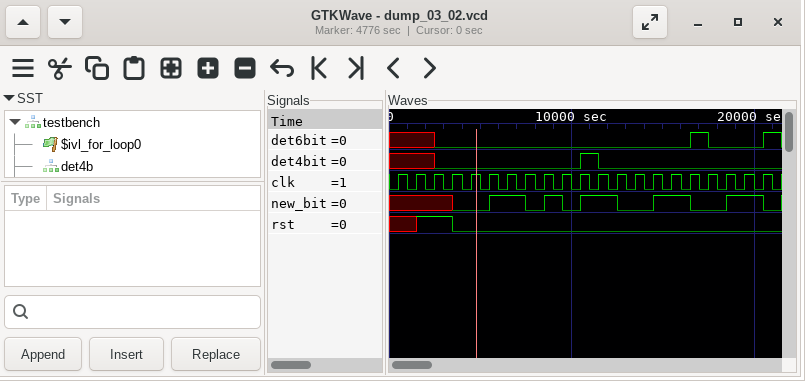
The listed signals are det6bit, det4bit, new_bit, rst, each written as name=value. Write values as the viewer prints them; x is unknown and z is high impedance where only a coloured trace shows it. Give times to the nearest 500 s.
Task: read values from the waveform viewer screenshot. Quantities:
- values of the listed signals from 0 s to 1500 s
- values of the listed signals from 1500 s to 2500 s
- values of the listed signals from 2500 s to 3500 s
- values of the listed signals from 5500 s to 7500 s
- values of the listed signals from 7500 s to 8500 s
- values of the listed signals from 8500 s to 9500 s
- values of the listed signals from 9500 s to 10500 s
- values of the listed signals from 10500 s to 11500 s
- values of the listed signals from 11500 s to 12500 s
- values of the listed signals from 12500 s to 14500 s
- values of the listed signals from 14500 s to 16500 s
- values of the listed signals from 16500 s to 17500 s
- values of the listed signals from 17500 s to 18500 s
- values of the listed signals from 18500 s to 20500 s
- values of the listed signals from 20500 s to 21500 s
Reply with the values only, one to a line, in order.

det6bit=x, det4bit=x, new_bit=x, rst=x
det6bit=x, det4bit=x, new_bit=x, rst=1
det6bit=0, det4bit=0, new_bit=x, rst=1
det6bit=0, det4bit=0, new_bit=1, rst=0
det6bit=0, det4bit=0, new_bit=0, rst=0
det6bit=0, det4bit=0, new_bit=1, rst=0
det6bit=0, det4bit=0, new_bit=0, rst=0
det6bit=0, det4bit=1, new_bit=1, rst=0
det6bit=0, det4bit=0, new_bit=1, rst=0
det6bit=0, det4bit=0, new_bit=0, rst=0
det6bit=0, det4bit=0, new_bit=1, rst=0
det6bit=1, det4bit=0, new_bit=0, rst=0
det6bit=0, det4bit=0, new_bit=0, rst=0
det6bit=0, det4bit=0, new_bit=1, rst=0
det6bit=1, det4bit=0, new_bit=0, rst=0
